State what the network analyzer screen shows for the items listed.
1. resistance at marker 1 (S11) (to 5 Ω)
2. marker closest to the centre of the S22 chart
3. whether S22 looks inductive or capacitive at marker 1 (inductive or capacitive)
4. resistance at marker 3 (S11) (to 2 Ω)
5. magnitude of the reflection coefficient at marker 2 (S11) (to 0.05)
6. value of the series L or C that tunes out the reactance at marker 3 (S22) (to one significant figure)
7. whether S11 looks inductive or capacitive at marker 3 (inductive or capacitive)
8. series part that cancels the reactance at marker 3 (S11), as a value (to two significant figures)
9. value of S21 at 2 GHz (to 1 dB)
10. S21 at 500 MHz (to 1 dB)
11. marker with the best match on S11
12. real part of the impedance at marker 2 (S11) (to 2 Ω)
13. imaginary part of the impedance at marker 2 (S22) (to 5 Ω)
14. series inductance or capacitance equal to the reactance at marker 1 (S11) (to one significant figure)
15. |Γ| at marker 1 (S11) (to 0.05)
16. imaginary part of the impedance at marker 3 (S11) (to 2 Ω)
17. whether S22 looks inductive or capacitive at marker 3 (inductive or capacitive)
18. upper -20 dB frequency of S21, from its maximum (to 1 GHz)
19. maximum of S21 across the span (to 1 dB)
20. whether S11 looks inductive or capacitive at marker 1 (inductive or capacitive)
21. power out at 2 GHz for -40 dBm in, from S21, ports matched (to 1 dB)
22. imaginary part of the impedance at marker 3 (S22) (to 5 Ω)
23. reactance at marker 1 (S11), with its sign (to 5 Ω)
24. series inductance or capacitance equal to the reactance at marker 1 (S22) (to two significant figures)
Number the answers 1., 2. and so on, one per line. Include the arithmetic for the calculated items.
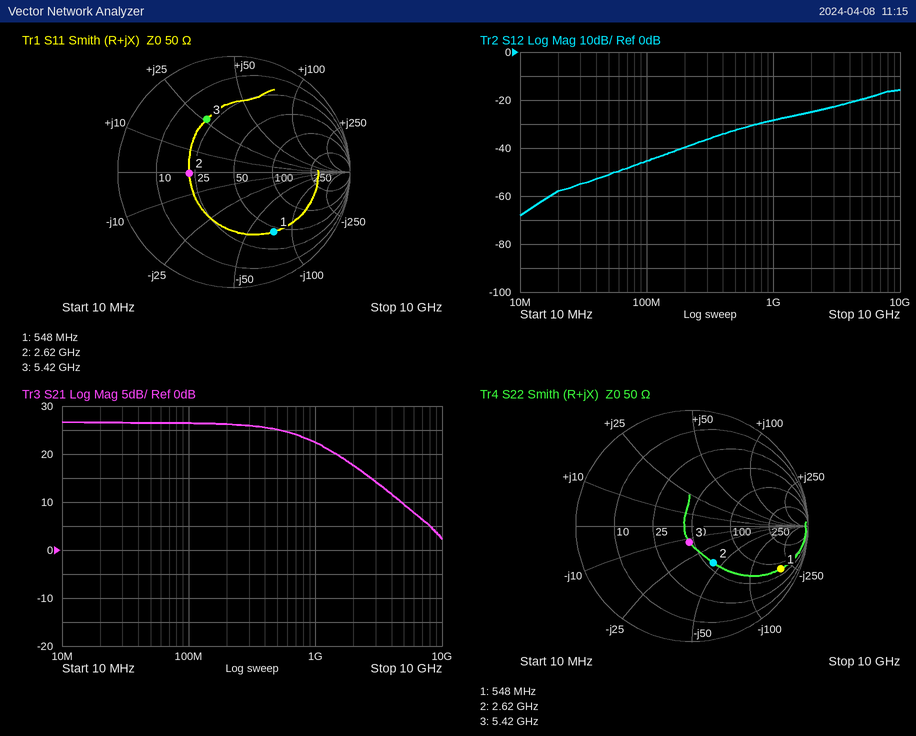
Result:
1. 45 Ω
2. marker 3
3. capacitive
4. 22 Ω
5. 0.40
6. L = 15 Ω/(2π × 5.42 GHz) ≈ 440 pH, so 400 pH to one significant figure
7. inductive
8. C = 1/(2π × 5.42 GHz × 26 Ω) ≈ 1.1 pF
9. 18 dB
10. 25 dB
11. marker 2
12. 22 Ω
13. -40 Ω
14. C = 1/(2π × 548 MHz × 75 Ω) ≈ 4 pF
15. 0.60
16. +26 Ω
17. capacitive
18. 7 GHz
19. 27 dB
20. capacitive
21. -40 dBm + (18 dB) = -22 dBm
22. -15 Ω
23. -75 Ω
24. C = 1/(2π × 548 MHz × 200 Ω) ≈ 1.5 pF
